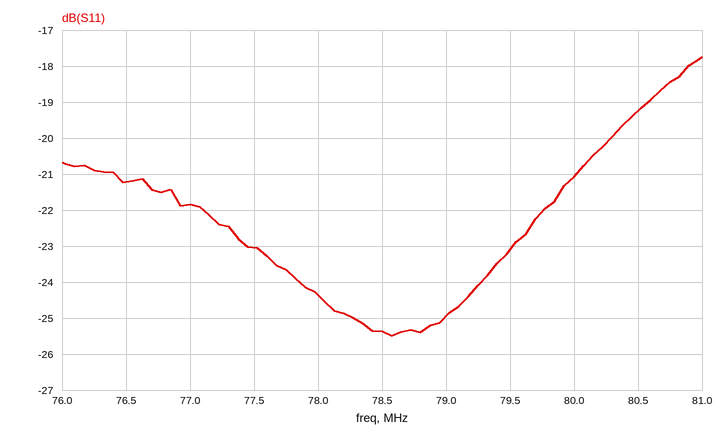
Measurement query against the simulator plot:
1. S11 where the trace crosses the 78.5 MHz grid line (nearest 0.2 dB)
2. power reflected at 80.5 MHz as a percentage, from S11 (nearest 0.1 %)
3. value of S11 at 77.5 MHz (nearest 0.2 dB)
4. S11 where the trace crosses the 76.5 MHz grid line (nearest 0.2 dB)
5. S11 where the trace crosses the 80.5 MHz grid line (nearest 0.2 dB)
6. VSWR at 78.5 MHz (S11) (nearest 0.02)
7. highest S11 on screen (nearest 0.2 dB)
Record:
-25.4 dB
1.2 %
-23.0 dB
-21.2 dB
-19.2 dB
1.12
-17.8 dB
